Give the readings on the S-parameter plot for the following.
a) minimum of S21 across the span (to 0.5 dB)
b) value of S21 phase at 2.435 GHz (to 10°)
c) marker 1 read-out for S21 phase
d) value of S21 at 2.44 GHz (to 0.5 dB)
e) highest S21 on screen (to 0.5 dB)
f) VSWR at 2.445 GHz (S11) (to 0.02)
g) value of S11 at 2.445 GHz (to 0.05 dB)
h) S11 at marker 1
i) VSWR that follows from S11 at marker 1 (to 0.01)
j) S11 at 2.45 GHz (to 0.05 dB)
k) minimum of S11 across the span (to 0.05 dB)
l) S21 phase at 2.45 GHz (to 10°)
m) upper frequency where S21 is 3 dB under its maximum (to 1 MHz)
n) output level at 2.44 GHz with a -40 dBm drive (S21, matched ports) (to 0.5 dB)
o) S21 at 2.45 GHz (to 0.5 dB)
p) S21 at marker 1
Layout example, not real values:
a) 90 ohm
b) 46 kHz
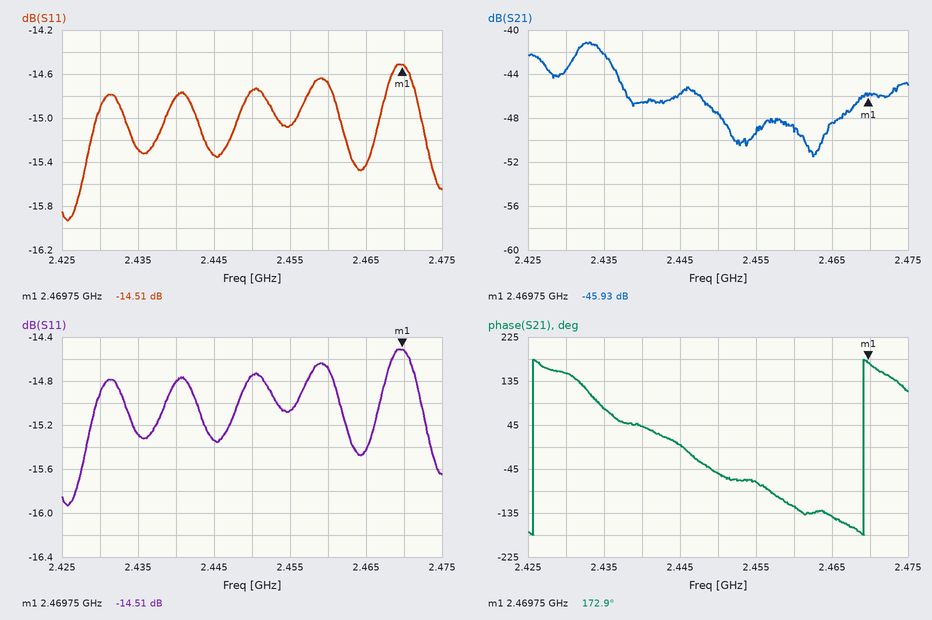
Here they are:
a) -51.5 dB
b) 80°
c) 172.9°
d) -46.5 dB
e) -41.0 dB
f) 1.42
g) -15.35 dB
h) -14.51 dB
i) 1.46
j) -14.75 dB
k) -15.95 dB
l) -50°
m) 2.437 GHz
n) -86.5 dBm
o) -47.5 dB
p) -45.93 dB
